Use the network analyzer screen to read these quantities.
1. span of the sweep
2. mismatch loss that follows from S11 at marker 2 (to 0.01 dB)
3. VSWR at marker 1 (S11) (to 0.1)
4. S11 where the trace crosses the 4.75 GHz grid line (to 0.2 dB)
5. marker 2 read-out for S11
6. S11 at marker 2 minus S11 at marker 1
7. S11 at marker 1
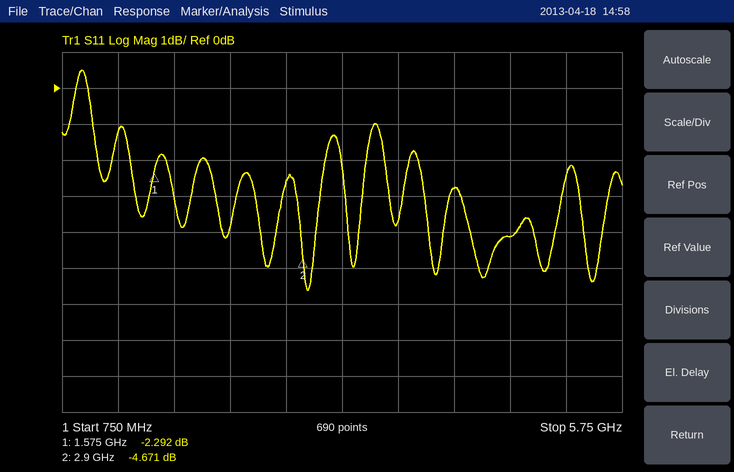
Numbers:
5 GHz
1.81 dB
7.6
-4.2 dB
-4.671 dB
-2.379 dB
-2.292 dB
